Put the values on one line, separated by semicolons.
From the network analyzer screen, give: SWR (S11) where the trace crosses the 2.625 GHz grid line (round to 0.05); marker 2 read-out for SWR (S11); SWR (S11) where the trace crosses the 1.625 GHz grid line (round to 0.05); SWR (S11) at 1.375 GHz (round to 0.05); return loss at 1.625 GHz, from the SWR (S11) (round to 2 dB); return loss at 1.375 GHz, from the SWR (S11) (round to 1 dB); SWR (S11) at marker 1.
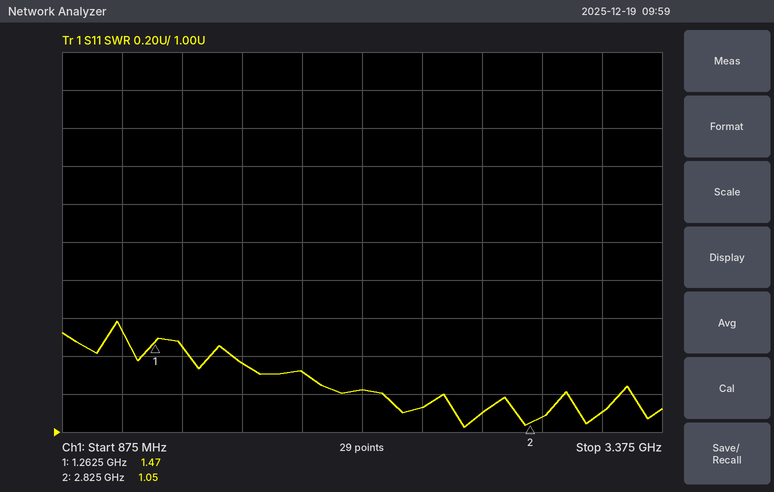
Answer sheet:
1.10; 1.05; 1.35; 1.45; 16 dB; 15 dB; 1.47
